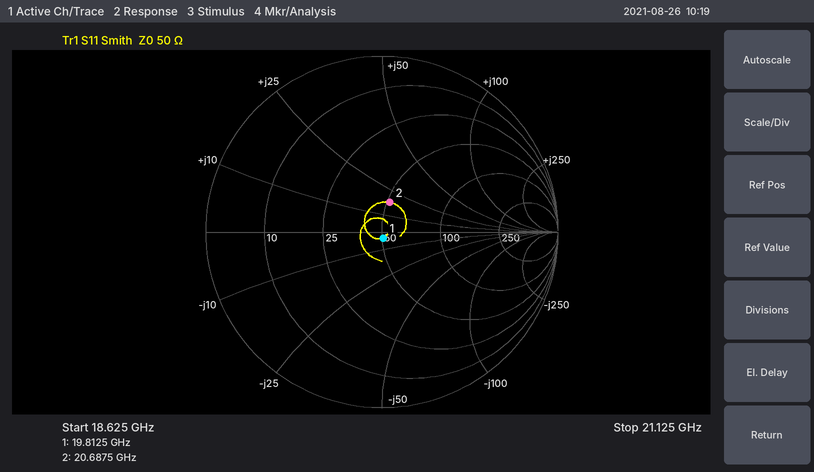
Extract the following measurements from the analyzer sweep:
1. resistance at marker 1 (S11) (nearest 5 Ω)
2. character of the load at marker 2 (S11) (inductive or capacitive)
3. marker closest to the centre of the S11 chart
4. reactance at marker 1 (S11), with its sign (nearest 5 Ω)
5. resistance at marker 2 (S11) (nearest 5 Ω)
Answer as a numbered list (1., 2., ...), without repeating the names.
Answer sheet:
1. 50 Ω
2. inductive
3. marker 1
4. -5 Ω
5. 50 Ω
